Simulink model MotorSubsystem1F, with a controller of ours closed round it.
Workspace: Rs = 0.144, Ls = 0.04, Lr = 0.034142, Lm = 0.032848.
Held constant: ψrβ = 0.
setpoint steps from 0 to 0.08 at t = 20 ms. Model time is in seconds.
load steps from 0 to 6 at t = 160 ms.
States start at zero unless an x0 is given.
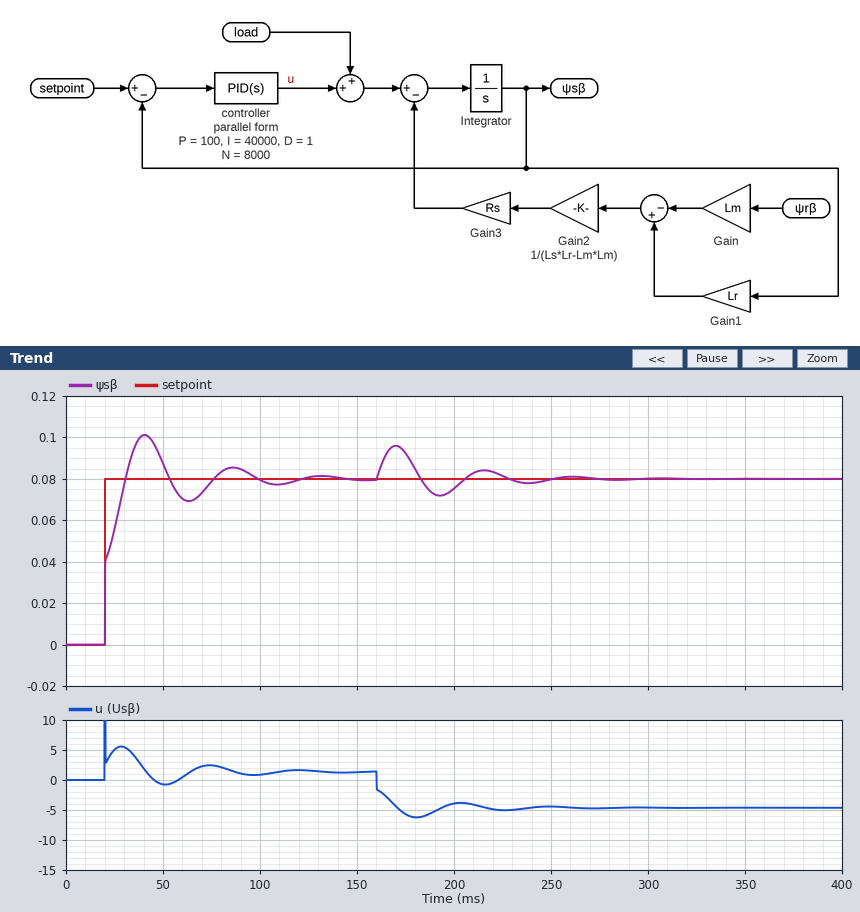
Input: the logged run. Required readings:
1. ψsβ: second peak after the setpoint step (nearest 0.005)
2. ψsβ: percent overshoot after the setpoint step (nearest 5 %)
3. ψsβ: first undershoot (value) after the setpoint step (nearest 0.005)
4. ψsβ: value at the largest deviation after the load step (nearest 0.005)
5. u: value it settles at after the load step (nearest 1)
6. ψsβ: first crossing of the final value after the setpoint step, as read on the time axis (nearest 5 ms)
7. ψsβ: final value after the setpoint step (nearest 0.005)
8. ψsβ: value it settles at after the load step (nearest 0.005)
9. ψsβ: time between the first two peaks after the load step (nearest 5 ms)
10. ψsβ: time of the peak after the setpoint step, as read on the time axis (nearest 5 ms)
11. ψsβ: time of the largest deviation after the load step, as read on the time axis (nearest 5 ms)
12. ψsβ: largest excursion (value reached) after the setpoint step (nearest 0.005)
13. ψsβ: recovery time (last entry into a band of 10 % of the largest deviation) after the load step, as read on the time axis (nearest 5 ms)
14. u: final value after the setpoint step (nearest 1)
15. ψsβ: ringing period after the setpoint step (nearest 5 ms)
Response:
0.085
25 %
0.070
0.095
-5
30 ms
0.080
0.080
45 ms
40 ms
170 ms
0.100
245 ms
1
45 ms
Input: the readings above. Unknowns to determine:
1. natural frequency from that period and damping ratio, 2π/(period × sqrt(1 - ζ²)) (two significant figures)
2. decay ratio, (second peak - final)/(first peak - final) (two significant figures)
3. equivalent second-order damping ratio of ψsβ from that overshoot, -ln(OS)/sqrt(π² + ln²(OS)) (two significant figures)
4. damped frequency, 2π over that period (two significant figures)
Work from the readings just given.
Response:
0.15 rad/ms
0.25
0.40
0.14 rad/ms
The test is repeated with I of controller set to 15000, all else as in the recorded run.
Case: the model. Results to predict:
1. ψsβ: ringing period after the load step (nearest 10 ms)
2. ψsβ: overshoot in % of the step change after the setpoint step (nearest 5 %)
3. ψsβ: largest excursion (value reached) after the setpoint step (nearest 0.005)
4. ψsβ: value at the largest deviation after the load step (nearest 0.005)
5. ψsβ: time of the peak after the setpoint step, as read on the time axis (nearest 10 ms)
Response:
80 ms
20 %
0.095
0.100
50 ms
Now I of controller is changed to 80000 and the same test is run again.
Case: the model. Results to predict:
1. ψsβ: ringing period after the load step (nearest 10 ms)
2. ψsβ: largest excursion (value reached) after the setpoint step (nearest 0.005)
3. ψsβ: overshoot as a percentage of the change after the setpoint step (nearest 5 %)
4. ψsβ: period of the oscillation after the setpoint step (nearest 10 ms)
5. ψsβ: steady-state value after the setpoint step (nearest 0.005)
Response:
30 ms
0.105
30 %
30 ms
0.080
